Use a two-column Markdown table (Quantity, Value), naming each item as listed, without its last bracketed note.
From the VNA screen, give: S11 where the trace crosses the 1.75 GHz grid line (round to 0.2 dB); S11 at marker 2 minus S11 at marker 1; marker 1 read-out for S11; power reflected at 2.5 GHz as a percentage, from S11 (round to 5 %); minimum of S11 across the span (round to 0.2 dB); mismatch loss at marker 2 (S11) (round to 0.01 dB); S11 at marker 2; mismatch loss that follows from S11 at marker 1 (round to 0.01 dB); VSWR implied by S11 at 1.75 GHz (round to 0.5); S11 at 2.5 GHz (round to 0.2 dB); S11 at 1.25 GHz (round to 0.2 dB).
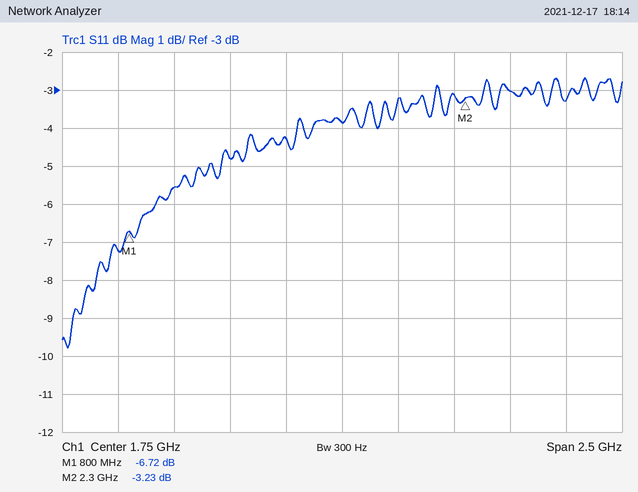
| Quantity | Value |
|---|---|
| S11 where the trace crosses the 1.75 GHz grid line | -3.8 dB |
| S11 at marker 2 minus S11 at marker 1 | 3.49 dB |
| marker 1 read-out for S11 | -6.72 dB |
| power reflected at 2.5 GHz as a percentage, from S11 | 50 % |
| minimum of S11 across the span | -9.8 dB |
| mismatch loss at marker 2 (S11) | 2.80 dB |
| S11 at marker 2 | -3.23 dB |
| mismatch loss that follows from S11 at marker 1 | 1.04 dB |
| VSWR implied by S11 at 1.75 GHz | 4.5 |
| S11 at 2.5 GHz | -3.0 dB |
| S11 at 1.25 GHz | -4.8 dB |
